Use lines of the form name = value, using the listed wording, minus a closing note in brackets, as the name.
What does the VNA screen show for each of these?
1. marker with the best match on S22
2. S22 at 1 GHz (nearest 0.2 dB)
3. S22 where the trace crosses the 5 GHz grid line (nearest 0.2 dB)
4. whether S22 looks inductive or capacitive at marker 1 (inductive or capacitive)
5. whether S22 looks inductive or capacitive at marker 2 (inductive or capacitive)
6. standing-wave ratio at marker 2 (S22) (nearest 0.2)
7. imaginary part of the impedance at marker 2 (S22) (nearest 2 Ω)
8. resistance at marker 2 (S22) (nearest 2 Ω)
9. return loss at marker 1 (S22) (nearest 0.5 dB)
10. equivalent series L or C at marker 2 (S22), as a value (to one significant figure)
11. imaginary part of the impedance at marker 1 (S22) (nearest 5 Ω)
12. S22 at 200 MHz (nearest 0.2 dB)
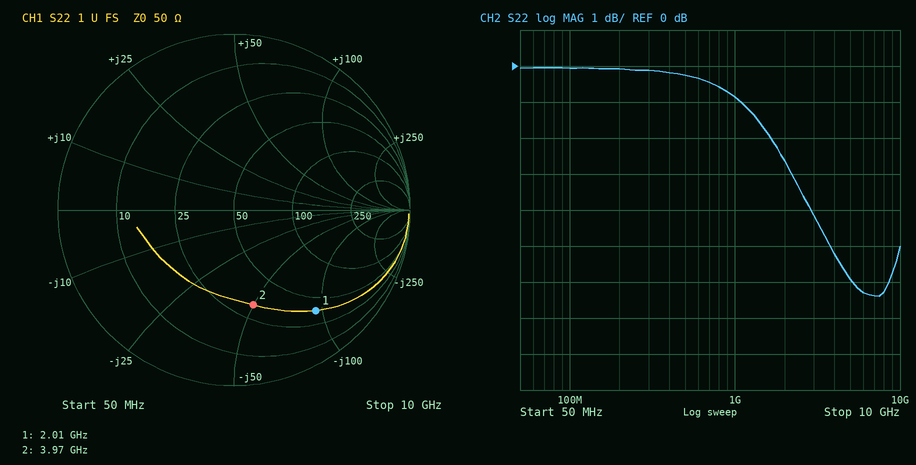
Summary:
marker with the best match on S22 = marker 2
S22 at 1 GHz = -0.8 dB
S22 where the trace crosses the 5 GHz grid line = -6.0 dB
whether S22 looks inductive or capacitive at marker 1 = capacitive
whether S22 looks inductive or capacitive at marker 2 = capacitive
standing-wave ratio at marker 2 (S22) = 3.4
imaginary part of the impedance at marker 2 (S22) = -50 Ω
resistance at marker 2 (S22) = 32 Ω
return loss at marker 1 (S22) = 2.5 dB
equivalent series L or C at marker 2 (S22), as a value = 800 fF
imaginary part of the impedance at marker 1 (S22) = -95 Ω
S22 at 200 MHz = 0.0 dB
